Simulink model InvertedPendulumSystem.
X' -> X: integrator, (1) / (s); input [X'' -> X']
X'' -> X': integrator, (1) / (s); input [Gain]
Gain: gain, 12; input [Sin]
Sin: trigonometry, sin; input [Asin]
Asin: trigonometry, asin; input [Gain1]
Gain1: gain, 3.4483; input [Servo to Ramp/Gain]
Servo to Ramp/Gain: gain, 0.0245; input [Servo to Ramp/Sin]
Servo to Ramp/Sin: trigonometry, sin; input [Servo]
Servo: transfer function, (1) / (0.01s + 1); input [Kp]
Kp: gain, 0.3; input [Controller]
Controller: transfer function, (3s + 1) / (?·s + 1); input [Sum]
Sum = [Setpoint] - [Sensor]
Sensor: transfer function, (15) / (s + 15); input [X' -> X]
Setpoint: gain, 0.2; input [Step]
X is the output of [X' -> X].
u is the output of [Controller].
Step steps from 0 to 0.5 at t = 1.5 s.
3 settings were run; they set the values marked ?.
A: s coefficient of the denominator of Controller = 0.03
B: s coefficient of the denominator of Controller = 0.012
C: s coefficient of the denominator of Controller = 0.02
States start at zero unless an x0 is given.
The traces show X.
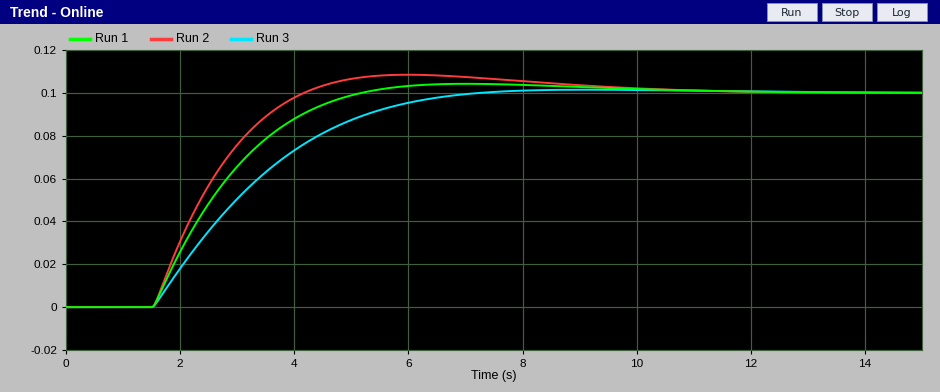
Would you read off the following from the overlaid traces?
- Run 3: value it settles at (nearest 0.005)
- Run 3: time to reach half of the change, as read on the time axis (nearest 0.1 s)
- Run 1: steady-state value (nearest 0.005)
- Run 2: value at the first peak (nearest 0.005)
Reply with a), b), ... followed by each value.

a) 0.100
b) 3.0 s
c) 0.100
d) 0.110
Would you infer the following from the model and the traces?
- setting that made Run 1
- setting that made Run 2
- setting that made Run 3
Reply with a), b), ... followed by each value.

a) C
b) A
c) B
